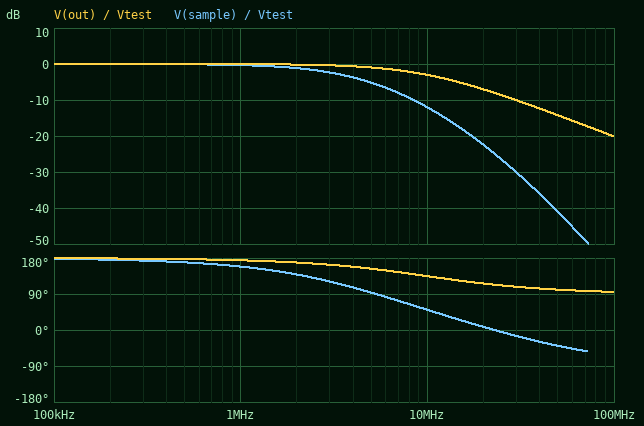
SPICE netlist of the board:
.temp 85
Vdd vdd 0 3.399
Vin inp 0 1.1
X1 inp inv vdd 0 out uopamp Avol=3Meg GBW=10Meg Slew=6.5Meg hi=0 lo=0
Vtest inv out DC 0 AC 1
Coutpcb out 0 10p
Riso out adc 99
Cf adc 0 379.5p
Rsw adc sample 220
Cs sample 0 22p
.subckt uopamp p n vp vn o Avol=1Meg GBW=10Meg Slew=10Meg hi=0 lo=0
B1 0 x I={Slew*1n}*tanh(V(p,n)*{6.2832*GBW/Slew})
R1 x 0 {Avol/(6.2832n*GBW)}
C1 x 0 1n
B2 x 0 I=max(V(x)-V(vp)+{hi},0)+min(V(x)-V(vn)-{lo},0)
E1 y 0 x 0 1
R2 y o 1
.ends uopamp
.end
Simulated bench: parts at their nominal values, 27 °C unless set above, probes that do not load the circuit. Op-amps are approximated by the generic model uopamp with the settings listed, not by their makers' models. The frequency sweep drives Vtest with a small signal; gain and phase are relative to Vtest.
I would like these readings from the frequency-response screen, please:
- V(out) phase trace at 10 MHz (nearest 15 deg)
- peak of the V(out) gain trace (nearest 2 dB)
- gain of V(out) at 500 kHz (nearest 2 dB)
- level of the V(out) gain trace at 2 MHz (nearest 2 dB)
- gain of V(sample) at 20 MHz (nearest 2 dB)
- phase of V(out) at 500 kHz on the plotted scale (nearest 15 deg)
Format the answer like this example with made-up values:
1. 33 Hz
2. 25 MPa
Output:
1. 135 deg
2. 0 dB
3. 0 dB
4. 0 dB
5. -22 dB
6. 180 deg
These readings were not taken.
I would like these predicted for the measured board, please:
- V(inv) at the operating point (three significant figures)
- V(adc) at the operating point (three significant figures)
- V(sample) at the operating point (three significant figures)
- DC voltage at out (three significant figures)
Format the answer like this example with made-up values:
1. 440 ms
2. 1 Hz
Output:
1. 1.10 V
2. 1.10 V
3. 1.10 V
4. 1.10 V
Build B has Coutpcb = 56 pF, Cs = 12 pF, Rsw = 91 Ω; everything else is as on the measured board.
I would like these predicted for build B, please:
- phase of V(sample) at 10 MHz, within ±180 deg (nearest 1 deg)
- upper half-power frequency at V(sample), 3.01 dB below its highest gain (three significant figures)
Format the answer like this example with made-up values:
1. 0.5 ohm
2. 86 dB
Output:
1. 63 deg
2. 3.61 MHz
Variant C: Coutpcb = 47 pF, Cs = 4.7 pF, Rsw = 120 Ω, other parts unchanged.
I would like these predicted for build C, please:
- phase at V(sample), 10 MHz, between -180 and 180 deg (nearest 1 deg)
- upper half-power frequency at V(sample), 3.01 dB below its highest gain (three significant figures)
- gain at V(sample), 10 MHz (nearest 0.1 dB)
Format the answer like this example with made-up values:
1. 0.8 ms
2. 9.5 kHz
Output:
1. 65 deg
2. 3.67 MHz
3. -11.3 dB
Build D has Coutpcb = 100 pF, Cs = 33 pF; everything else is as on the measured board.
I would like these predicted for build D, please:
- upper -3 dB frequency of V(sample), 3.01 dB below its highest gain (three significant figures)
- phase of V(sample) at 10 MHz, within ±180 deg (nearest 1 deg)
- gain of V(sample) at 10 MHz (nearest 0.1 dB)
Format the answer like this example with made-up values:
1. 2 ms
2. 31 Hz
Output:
1. 3.36 MHz
2. 43 deg
3. -12.6 dB
